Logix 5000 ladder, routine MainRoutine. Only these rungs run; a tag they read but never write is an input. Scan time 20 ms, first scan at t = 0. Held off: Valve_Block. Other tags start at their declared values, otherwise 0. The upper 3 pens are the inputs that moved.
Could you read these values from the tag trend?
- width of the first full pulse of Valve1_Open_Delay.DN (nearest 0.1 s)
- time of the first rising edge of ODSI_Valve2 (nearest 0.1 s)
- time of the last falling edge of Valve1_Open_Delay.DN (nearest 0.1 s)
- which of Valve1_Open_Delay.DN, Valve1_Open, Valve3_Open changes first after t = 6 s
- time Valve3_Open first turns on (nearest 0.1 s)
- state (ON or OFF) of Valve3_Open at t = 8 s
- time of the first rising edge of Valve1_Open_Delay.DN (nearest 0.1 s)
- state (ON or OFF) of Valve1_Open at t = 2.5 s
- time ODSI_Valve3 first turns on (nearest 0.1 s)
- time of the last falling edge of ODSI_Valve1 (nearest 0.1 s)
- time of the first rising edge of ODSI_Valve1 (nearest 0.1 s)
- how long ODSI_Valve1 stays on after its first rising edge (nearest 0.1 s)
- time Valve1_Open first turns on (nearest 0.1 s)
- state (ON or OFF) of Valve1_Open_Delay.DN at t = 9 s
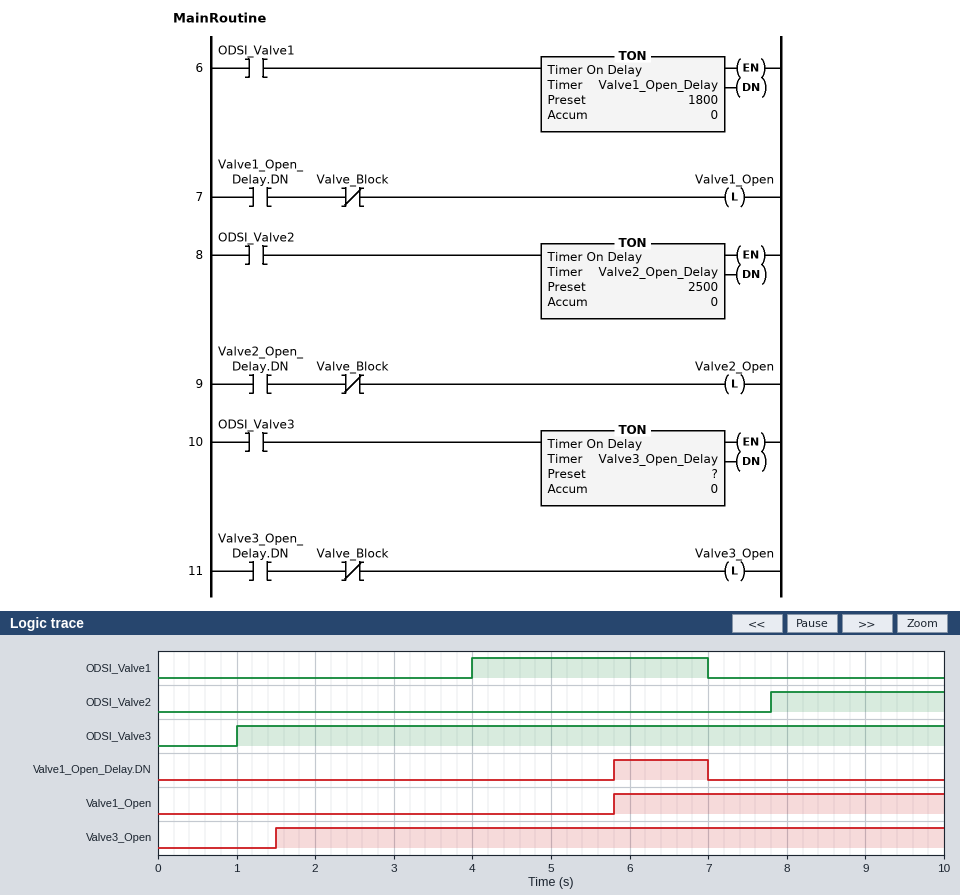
1.2 s
7.8 s
7.0 s
Valve1_Open_Delay.DN
1.5 s
ON
5.8 s
OFF
1.0 s
7.0 s
4.0 s
3.0 s
5.8 s
OFF
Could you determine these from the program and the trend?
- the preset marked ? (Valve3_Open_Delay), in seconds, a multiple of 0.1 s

0.5 s
